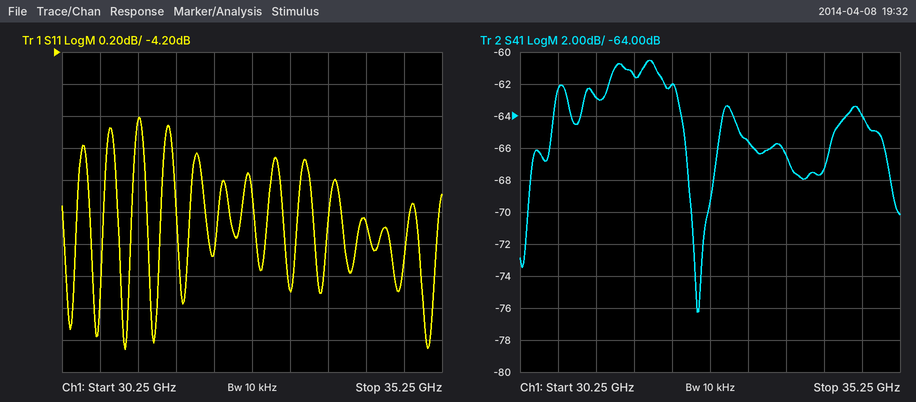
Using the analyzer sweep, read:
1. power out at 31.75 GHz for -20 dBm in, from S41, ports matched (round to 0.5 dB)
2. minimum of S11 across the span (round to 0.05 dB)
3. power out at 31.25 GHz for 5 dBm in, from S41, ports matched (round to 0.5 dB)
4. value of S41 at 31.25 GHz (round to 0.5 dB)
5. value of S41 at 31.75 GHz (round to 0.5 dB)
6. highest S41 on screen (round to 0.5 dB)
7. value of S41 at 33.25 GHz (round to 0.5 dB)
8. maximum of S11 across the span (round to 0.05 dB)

-81.5 dBm
-6.05 dB
-58.0 dBm
-63.0 dB
-61.5 dB
-60.5 dB
-65.5 dB
-4.60 dB
